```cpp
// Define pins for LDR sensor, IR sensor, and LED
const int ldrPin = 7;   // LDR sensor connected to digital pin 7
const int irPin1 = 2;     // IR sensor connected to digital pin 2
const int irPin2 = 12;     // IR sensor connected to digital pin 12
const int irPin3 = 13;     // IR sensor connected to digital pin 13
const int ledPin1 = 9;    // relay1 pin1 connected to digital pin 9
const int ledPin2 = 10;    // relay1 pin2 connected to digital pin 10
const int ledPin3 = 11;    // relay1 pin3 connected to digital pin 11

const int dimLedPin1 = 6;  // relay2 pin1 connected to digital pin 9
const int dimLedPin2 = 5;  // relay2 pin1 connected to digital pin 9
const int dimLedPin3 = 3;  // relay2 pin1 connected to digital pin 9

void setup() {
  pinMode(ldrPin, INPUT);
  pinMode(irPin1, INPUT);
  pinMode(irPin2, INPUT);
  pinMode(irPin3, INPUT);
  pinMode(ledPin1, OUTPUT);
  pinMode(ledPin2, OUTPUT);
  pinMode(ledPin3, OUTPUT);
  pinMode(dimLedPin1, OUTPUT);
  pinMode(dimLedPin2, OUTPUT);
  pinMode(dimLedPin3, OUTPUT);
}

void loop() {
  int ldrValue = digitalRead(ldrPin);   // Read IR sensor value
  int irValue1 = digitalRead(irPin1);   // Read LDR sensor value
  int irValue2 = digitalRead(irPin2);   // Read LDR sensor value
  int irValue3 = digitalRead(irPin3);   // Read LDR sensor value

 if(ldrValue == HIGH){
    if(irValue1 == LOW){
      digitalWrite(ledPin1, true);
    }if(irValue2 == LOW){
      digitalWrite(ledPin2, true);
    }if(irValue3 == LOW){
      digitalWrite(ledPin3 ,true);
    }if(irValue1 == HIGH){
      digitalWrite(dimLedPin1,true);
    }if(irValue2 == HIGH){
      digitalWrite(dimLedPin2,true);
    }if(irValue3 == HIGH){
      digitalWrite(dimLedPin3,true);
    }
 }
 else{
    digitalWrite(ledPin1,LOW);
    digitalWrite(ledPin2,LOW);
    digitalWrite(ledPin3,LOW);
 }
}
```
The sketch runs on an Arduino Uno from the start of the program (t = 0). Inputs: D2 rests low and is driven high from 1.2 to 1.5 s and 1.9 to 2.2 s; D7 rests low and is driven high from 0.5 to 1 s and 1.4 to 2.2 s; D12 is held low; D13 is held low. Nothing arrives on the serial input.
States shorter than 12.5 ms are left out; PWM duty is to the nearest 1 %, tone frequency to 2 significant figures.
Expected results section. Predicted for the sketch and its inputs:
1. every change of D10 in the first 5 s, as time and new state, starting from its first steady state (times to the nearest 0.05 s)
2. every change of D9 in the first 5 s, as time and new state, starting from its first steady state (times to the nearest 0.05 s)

0 s low; 0.5 s high; 1 s low; 1.4 s high; 2.2 s low
0 s low; 0.5 s high; 1 s low; 1.5 s high; 2.2 s low
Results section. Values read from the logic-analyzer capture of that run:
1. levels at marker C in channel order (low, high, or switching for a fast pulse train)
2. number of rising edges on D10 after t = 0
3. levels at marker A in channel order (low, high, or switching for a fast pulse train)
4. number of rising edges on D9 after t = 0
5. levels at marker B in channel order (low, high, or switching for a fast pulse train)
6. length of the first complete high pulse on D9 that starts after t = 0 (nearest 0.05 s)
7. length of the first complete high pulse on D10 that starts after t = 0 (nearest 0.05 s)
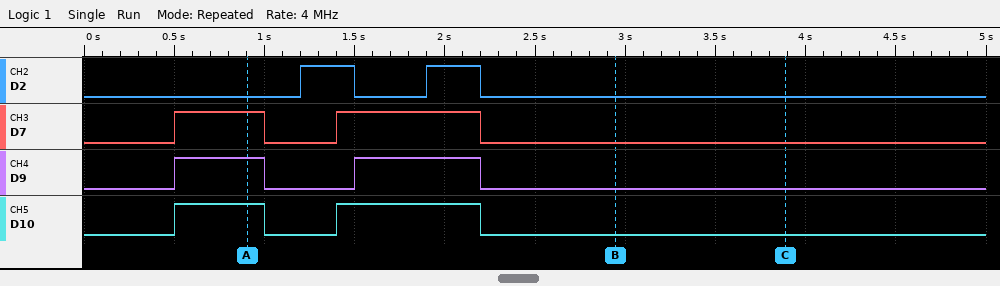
D2 low, D7 low, D9 low, D10 low
2
D2 low, D7 high, D9 high, D10 high
2
D2 low, D7 low, D9 low, D10 low
0.50 s
0.50 s
